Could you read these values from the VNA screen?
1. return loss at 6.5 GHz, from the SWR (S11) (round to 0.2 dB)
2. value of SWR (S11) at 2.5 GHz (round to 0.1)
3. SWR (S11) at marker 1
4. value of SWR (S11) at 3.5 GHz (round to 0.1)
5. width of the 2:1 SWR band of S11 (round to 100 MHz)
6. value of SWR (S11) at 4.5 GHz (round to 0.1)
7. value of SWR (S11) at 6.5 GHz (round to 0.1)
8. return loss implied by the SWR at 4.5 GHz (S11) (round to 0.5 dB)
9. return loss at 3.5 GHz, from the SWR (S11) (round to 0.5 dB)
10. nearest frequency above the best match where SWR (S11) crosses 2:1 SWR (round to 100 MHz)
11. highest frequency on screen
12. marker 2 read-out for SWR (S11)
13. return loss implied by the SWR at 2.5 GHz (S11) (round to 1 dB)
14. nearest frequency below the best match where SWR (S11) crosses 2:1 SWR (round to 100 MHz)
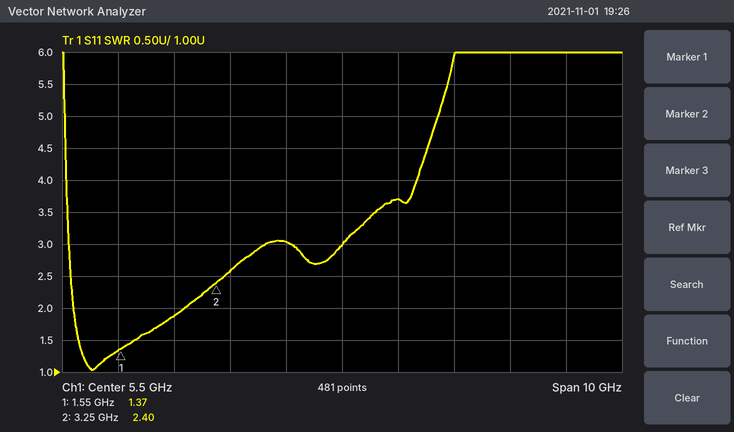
4.8 dB
1.9
1.37
2.6
2.0 GHz
3.0
3.7
6.0 dB
7.0 dB
2.7 GHz
10.5 GHz
2.40
10 dB
700 MHz
